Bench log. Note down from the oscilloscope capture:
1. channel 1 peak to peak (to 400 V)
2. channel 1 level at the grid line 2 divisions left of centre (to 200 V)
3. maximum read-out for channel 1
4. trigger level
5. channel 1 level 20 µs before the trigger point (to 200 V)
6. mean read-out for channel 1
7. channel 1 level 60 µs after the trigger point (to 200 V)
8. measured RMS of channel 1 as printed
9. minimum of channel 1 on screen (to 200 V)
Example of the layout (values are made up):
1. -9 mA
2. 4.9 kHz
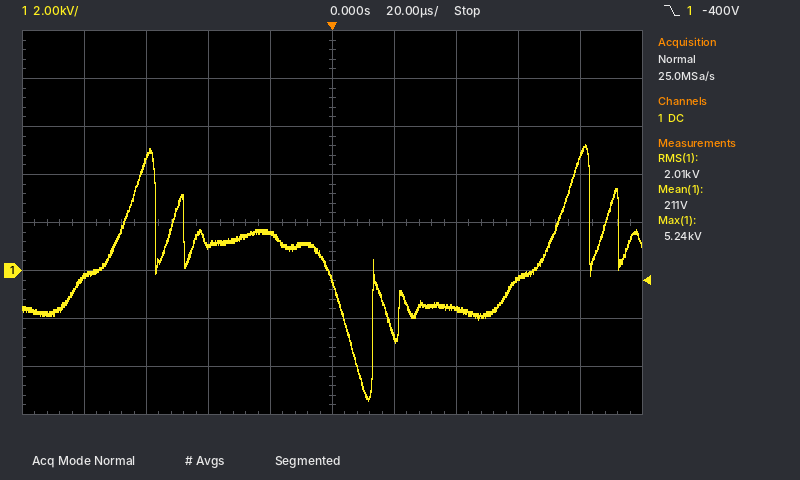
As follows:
1. 10.8 kV
2. 1.0 kV
3. 5.24 kV
4. -400 V
5. 1.6 kV
6. 211 V
7. -400 V
8. 2.01 kV
9. -5.4 kV
